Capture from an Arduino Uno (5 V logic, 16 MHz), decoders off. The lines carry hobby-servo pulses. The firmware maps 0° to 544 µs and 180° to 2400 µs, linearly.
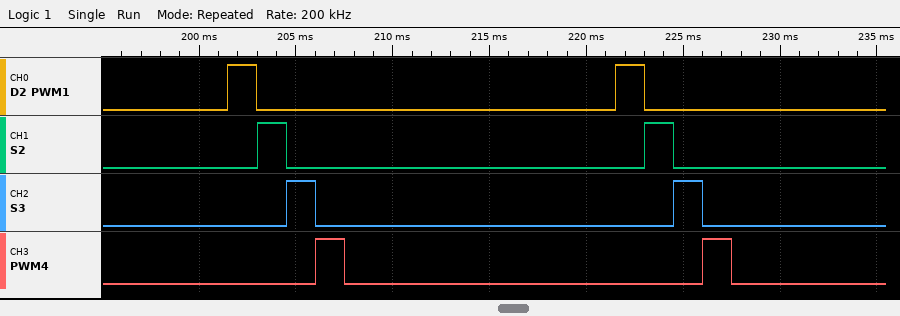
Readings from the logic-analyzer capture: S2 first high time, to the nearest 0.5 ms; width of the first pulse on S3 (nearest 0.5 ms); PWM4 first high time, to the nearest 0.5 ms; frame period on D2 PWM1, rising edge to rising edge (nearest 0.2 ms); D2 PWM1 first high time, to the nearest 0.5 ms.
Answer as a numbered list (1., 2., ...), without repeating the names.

1. 1.5 ms
2. 1.5 ms
3. 1.5 ms
4. 20.0 ms
5. 1.5 ms
